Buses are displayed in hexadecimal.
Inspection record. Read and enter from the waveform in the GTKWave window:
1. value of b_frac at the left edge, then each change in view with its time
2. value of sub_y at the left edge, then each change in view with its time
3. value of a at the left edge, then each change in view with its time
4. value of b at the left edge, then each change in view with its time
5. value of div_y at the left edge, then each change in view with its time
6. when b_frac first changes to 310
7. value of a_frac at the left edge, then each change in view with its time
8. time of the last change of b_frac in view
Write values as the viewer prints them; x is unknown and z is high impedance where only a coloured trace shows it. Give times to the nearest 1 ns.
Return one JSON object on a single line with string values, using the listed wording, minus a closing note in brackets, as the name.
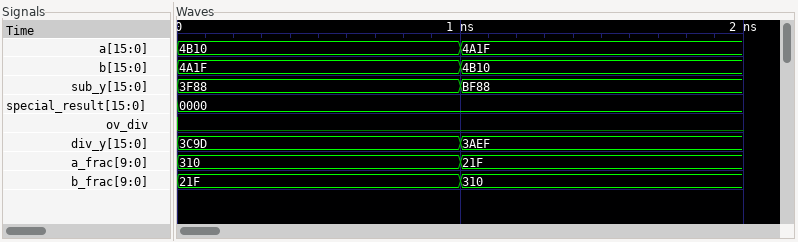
{"value of b_frac at the left edge, then each change in view with its time": "21F, 310 at 1 ns", "value of sub_y at the left edge, then each change in view with its time": "3F88, BF88 at 1 ns", "value of a at the left edge, then each change in view with its time": "4B10, 4A1F at 1 ns", "value of b at the left edge, then each change in view with its time": "4A1F, 4B10 at 1 ns", "value of div_y at the left edge, then each change in view with its time": "3C9D, 3AEF at 1 ns", "when b_frac first changes to 310": "1 ns", "value of a_frac at the left edge, then each change in view with its time": "310, 21F at 1 ns", "time of the last change of b_frac in view": "1 ns"}
